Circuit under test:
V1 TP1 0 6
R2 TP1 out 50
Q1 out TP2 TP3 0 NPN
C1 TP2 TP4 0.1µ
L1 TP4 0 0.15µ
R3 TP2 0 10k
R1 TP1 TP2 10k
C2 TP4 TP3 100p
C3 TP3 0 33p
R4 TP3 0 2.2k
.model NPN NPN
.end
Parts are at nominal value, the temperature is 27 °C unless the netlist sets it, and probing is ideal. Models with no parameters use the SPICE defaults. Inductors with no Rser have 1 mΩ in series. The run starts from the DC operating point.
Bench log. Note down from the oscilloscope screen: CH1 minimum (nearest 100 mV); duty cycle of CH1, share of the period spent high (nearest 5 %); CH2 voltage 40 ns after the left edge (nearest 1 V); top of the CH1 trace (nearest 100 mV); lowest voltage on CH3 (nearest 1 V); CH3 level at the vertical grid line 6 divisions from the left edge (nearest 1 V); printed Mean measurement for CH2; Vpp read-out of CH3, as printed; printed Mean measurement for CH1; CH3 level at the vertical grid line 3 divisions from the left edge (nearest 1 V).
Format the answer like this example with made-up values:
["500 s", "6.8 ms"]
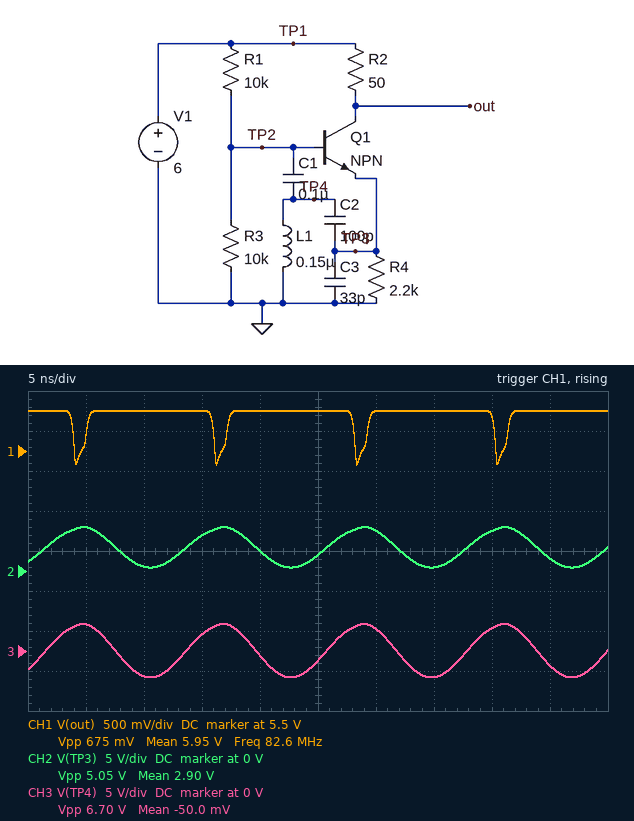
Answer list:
["5.3 V", "90 %", "5 V", "6.0 V", "-3 V", "3 V", "2.90 V", "6.70 V", "5.95 V", "2 V"]
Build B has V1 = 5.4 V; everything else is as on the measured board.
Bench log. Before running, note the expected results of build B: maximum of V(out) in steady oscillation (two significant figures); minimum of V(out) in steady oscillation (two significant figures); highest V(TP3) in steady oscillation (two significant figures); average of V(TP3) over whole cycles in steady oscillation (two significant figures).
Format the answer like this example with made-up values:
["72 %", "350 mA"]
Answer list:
["5.4 V", "4.8 V", "4.9 V", "2.6 V"]
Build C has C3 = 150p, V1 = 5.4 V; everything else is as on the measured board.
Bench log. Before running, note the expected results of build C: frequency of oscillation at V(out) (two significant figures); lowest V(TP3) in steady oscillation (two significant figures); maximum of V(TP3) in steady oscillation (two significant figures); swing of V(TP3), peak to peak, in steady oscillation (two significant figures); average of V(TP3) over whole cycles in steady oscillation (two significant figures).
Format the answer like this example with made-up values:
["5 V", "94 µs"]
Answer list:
["53 MHz", "2.3 V", "4.5 V", "2.2 V", "3.4 V"]
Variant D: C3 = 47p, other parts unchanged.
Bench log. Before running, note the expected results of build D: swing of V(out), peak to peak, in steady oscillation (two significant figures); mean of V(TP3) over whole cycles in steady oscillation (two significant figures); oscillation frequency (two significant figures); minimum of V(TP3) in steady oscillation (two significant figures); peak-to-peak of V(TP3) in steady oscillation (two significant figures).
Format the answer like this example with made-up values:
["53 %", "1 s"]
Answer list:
["730 mV", "3.1 V", "73 MHz", "910 mV", "4.5 V"]
